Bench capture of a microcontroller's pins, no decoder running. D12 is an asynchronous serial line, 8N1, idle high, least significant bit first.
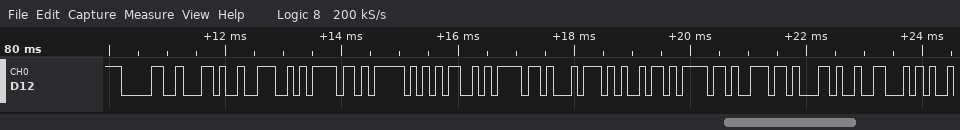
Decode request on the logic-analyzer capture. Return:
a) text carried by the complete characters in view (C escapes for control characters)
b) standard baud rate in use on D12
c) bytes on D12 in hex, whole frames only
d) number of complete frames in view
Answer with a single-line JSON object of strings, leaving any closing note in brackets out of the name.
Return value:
{"text carried by the complete characters in view": "\"0,No_Motion,F\"", "standard baud rate in use on D12": "9600 baud", "bytes on D12 in hex, whole frames only": "30 2C 4E 6F 5F 4D 6F 74 69 6F 6E 2C 46", "number of complete frames in view": "13"}
